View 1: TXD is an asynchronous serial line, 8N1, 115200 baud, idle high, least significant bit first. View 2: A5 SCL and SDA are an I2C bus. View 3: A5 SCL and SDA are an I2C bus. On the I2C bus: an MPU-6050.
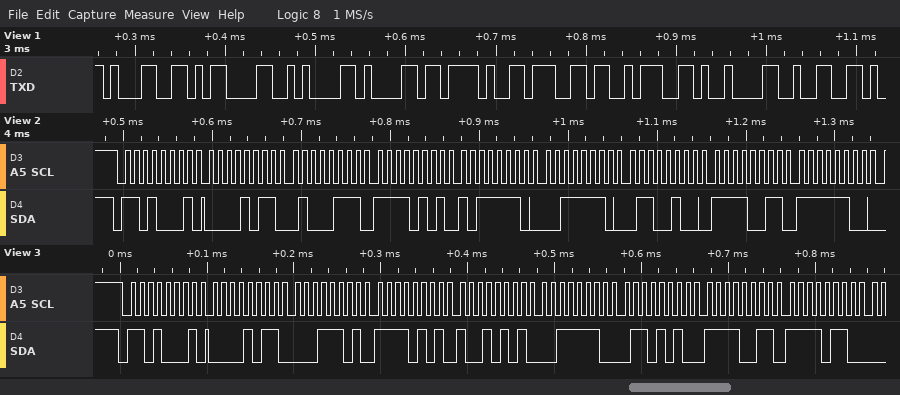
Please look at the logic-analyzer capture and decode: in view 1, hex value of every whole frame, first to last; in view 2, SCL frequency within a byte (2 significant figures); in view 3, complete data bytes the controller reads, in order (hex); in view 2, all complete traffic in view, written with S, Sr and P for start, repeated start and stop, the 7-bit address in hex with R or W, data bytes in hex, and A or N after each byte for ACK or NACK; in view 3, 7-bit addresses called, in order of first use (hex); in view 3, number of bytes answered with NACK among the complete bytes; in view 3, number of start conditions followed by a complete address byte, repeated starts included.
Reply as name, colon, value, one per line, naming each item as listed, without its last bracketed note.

in view 1, hex value of every whole frame, first to last: 31 0D 0A 61 2F 67 3A 09 32
in view 2, SCL frequency within a byte: 100 kHz
in view 3, complete data bytes the controller reads, in order: 0B 1D F5 95 3E 6A F3 F6
in view 2, all complete traffic in view, written with S, Sr and P for start, repeated start and stop, the 7-bit address in hex with R or W, data bytes in hex, and A or N after each byte for ACK or NACK: S 68R A 0B A 47 A F5 A BE A 3E A 64 A F3 A FC A
in view 3, 7-bit addresses called, in order of first use: 0x68
in view 3, number of bytes answered with NACK among the complete bytes: 0
in view 3, number of start conditions followed by a complete address byte, repeated starts included: 1
